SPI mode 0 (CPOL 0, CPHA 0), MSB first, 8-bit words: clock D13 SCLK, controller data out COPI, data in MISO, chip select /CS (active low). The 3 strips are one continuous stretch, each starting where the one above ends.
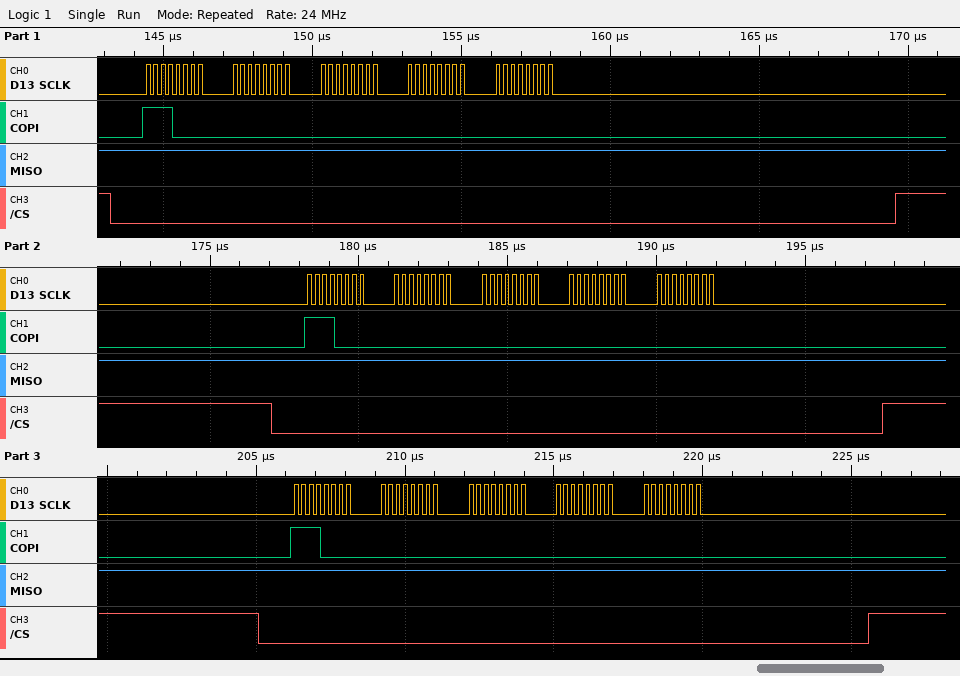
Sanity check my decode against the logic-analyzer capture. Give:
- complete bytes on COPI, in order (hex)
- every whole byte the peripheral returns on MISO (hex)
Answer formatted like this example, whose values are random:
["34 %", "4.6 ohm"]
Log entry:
["F0 00 00 00 00 F0 00 00 00 00 F0 00 00 00 00", "FF FF FF FF FF FF FF FF FF FF FF FF FF FF FF"]
